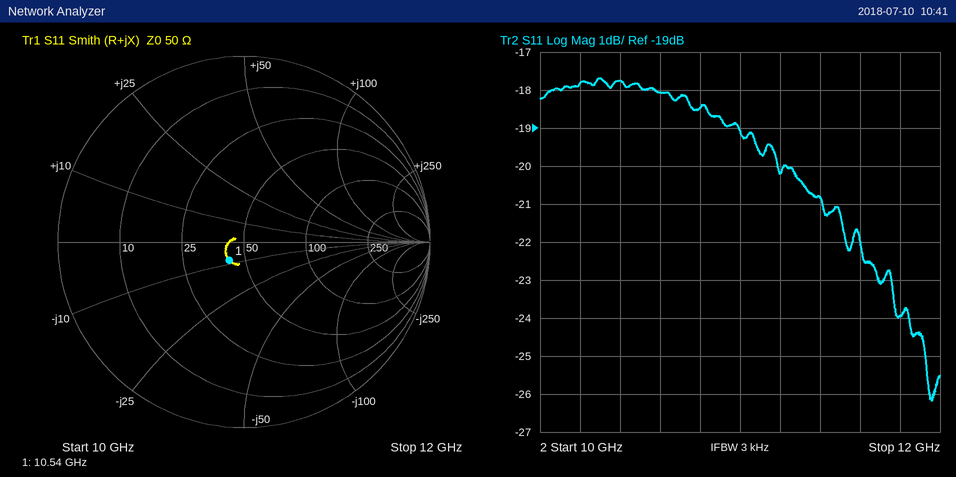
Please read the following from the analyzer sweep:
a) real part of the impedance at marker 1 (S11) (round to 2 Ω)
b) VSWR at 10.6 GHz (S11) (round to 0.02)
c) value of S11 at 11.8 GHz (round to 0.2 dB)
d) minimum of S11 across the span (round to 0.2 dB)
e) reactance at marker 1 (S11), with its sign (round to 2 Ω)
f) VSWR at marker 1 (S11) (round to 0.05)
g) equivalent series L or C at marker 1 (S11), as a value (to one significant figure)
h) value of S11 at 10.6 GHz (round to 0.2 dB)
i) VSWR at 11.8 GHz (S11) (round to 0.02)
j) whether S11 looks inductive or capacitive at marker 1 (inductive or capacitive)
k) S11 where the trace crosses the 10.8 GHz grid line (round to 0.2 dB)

42 Ω
1.28
-24.0 dB
-26.2 dB
-8 Ω
1.30
2 pF
-18.0 dB
1.14
capacitive
-18.4 dB
